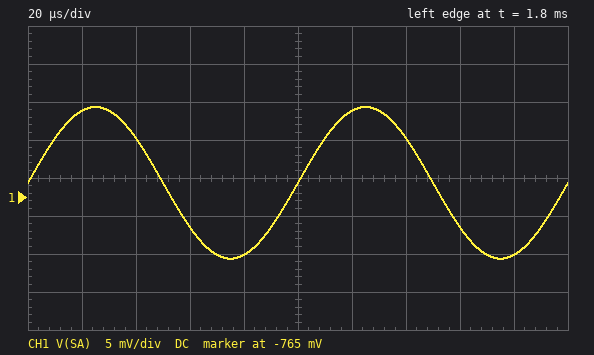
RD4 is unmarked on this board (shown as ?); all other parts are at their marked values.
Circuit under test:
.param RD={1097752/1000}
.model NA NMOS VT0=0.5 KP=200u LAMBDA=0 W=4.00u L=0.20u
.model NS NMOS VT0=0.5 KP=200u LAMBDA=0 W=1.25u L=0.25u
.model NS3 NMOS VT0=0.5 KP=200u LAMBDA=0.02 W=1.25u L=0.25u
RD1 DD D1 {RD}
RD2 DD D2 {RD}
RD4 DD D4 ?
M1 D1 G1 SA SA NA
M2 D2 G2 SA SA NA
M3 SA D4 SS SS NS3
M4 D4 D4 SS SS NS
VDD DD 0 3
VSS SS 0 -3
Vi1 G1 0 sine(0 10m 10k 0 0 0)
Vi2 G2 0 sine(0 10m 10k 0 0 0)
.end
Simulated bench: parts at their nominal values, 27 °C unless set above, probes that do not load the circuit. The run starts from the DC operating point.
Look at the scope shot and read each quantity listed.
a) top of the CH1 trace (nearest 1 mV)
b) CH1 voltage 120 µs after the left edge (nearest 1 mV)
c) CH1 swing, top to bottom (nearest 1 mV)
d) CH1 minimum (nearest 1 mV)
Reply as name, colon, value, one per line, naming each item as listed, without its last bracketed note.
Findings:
top of the CH1 trace: -753 mV
CH1 voltage 120 µs after the left edge: -754 mV
CH1 swing, top to bottom: 20 mV
CH1 minimum: -773 mV
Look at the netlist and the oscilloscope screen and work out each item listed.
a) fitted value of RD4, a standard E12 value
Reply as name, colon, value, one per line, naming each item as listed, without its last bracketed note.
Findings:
fitted value of RD4, a standard E12 value: 18 kΩ
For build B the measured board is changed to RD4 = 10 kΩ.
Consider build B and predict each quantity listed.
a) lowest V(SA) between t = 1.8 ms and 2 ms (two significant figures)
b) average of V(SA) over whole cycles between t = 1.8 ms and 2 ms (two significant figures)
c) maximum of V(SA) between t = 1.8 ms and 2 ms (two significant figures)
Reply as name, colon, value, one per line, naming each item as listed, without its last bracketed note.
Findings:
lowest V(SA) between t = 1.8 ms and 2 ms: -850 mV
average of V(SA) over whole cycles between t = 1.8 ms and 2 ms: -840 mV
maximum of V(SA) between t = 1.8 ms and 2 ms: -830 mV
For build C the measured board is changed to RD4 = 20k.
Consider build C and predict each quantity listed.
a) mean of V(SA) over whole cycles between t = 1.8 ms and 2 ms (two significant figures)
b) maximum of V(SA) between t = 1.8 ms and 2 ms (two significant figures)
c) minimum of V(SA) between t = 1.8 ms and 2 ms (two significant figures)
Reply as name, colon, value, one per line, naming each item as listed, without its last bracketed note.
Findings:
mean of V(SA) over whole cycles between t = 1.8 ms and 2 ms: -750 mV
maximum of V(SA) between t = 1.8 ms and 2 ms: -740 mV
minimum of V(SA) between t = 1.8 ms and 2 ms: -760 mV
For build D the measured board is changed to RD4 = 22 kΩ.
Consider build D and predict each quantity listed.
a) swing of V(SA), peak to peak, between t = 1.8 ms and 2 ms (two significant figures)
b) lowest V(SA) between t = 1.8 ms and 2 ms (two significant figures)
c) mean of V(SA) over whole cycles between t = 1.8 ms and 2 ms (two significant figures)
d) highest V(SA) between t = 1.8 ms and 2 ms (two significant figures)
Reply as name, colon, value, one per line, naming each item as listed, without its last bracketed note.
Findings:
swing of V(SA), peak to peak, between t = 1.8 ms and 2 ms: 20 mV
lowest V(SA) between t = 1.8 ms and 2 ms: -750 mV
mean of V(SA) over whole cycles between t = 1.8 ms and 2 ms: -740 mV
highest V(SA) between t = 1.8 ms and 2 ms: -730 mV
